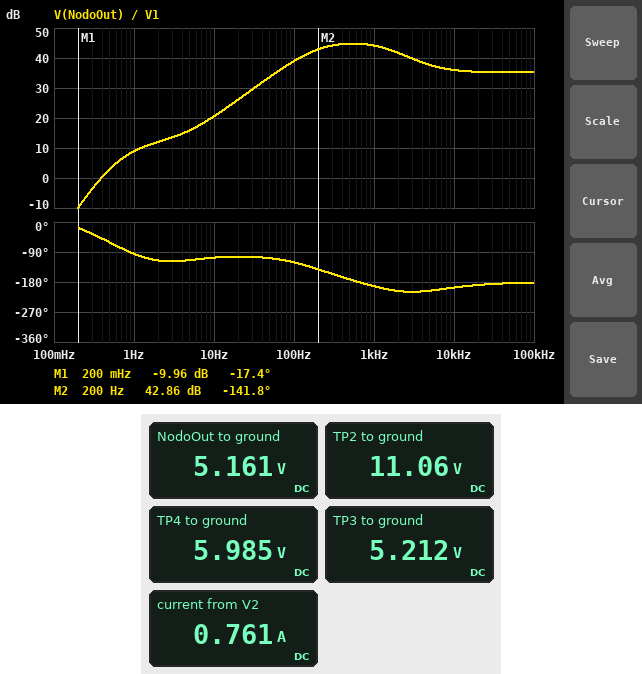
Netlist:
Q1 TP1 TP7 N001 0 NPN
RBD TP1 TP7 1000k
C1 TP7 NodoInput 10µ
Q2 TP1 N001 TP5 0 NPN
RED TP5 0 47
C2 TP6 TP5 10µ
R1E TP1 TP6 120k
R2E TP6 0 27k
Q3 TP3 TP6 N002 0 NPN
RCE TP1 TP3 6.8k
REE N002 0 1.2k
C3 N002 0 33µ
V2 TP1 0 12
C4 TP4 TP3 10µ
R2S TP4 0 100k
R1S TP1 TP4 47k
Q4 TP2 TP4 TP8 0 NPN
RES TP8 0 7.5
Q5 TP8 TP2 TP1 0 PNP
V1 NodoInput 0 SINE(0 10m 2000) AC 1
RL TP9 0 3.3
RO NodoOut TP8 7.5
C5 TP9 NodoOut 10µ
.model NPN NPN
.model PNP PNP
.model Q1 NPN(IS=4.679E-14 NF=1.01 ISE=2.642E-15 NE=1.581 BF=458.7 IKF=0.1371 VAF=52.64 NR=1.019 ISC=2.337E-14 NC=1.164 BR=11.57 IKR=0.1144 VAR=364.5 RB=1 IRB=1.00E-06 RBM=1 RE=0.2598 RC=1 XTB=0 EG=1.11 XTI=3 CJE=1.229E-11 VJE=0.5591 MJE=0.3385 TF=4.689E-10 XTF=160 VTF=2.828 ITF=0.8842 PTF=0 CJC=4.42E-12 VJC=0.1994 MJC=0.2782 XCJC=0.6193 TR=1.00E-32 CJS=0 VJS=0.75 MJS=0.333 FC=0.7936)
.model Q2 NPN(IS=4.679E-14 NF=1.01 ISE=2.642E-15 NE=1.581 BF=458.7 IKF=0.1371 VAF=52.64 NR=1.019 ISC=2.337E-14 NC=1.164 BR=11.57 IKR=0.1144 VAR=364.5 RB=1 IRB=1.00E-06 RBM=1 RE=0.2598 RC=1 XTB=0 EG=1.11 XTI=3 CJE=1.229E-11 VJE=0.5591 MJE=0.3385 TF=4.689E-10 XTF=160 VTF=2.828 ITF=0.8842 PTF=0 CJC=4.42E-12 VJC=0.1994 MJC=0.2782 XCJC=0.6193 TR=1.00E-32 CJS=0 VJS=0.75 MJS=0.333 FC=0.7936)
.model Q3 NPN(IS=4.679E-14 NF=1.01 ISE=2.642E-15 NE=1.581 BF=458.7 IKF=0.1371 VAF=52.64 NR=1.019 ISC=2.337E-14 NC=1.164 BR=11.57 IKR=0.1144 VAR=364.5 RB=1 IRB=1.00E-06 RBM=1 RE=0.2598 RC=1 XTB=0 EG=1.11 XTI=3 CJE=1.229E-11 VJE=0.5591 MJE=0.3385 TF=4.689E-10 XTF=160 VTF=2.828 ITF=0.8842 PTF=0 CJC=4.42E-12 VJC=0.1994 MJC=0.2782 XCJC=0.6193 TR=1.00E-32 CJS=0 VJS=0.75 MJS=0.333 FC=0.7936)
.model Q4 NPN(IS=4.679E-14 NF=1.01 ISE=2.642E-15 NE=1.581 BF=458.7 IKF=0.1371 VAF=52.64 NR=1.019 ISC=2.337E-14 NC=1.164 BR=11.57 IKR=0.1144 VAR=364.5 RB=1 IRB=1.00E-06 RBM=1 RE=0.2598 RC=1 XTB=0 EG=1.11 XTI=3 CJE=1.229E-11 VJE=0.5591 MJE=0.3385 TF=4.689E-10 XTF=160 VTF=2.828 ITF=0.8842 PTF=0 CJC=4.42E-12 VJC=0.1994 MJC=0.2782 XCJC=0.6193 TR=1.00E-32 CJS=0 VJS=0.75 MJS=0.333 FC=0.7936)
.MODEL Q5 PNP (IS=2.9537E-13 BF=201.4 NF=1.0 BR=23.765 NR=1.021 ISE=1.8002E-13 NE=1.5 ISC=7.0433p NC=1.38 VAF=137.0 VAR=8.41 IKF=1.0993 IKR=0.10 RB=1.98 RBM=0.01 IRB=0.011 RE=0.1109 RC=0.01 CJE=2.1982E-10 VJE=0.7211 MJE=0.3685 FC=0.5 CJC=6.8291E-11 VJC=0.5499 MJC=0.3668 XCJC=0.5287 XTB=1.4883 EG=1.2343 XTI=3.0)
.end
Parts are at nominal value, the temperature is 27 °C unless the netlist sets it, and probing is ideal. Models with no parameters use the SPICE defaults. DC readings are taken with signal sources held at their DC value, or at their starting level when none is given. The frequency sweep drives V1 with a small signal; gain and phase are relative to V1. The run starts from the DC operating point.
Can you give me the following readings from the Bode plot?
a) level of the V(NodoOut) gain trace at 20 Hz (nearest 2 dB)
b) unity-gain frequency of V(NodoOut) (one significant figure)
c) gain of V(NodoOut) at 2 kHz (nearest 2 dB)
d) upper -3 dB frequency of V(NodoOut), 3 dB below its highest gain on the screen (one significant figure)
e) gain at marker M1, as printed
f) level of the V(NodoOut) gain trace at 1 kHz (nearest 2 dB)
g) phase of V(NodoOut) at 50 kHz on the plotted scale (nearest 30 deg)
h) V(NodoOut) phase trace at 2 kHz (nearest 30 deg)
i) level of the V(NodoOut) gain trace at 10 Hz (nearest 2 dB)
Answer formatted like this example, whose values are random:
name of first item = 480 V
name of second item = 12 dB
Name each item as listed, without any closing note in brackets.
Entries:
level of the V(NodoOut) gain trace at 20 Hz = 26 dB
unity-gain frequency of V(NodoOut) = 400 mHz
gain of V(NodoOut) at 2 kHz = 42 dB
upper -3 dB frequency of V(NodoOut), 3 dB below its highest gain on the screen = 2 kHz
gain at marker M1, as printed = -9.96 dB
level of the V(NodoOut) gain trace at 1 kHz = 44 dB
phase of V(NodoOut) at 50 kHz on the plotted scale = -180 deg
V(NodoOut) phase trace at 2 kHz = -210 deg
level of the V(NodoOut) gain trace at 10 Hz = 20 dB
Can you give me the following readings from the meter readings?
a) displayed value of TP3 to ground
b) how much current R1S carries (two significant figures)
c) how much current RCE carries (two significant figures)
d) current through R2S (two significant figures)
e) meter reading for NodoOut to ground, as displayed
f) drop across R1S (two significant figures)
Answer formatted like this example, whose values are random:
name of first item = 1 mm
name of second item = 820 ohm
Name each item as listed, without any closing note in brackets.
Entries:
displayed value of TP3 to ground = 5.212 V
how much current R1S carries = 130 µA
how much current RCE carries = 1.0 mA
current through R2S = 60 µA
meter reading for NodoOut to ground, as displayed = 5.161 V
drop across R1S = 6.0 V
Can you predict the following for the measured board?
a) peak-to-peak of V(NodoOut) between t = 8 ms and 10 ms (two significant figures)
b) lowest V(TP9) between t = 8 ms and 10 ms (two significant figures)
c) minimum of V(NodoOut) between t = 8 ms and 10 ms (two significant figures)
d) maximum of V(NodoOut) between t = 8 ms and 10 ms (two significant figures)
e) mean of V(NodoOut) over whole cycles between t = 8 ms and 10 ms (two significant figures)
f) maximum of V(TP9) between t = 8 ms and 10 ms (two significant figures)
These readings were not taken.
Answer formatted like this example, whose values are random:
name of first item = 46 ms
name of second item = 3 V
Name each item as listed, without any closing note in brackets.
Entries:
peak-to-peak of V(NodoOut) between t = 8 ms and 10 ms = 2.4 V
lowest V(TP9) between t = 8 ms and 10 ms = -500 mV
minimum of V(NodoOut) between t = 8 ms and 10 ms = 3.9 V
maximum of V(NodoOut) between t = 8 ms and 10 ms = 6.3 V
mean of V(NodoOut) over whole cycles between t = 8 ms and 10 ms = 5.2 V
maximum of V(TP9) between t = 8 ms and 10 ms = 430 mV
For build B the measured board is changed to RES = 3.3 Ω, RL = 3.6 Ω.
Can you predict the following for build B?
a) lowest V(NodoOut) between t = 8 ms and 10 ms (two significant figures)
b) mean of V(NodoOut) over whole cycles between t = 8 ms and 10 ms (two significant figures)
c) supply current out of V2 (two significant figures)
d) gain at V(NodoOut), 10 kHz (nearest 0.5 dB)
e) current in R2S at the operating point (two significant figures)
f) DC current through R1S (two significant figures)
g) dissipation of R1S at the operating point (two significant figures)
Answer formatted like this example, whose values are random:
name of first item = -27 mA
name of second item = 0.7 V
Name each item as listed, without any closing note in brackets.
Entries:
lowest V(NodoOut) between t = 8 ms and 10 ms = 2.6 V
mean of V(NodoOut) over whole cycles between t = 8 ms and 10 ms = 3.7 V
supply current out of V2 = 1.2 A
gain at V(NodoOut), 10 kHz = 35.5 dB
current in R2S at the operating point = 46 µA
DC current through R1S = 160 µA
dissipation of R1S at the operating point = 1.2 mW
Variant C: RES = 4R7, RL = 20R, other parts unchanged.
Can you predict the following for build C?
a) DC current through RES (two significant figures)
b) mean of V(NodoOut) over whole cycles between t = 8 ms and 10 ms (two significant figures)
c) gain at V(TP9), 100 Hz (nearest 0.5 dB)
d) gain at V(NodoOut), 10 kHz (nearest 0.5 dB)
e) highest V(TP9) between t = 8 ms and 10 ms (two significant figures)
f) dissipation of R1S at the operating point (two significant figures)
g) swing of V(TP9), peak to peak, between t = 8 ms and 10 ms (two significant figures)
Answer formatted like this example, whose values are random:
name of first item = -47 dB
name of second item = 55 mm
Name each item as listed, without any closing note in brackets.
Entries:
DC current through RES = 930 mA
mean of V(NodoOut) over whole cycles between t = 8 ms and 10 ms = 4.4 V
gain at V(TP9), 100 Hz = 20.5 dB
gain at V(NodoOut), 10 kHz = 42.5 dB
highest V(TP9) between t = 8 ms and 10 ms = 1.2 V
dissipation of R1S at the operating point = 980 µW
swing of V(TP9), peak to peak, between t = 8 ms and 10 ms = 2.6 V
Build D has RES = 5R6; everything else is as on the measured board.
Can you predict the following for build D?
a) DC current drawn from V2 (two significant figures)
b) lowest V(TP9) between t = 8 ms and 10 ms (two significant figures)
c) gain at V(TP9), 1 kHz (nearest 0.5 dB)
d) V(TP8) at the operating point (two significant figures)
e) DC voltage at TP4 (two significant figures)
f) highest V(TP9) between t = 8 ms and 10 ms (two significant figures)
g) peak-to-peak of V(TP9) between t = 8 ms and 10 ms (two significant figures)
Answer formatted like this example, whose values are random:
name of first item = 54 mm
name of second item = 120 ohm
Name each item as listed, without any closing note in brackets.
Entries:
DC current drawn from V2 = 910 mA
lowest V(TP9) between t = 8 ms and 10 ms = -490 mV
gain at V(TP9), 1 kHz = 30.0 dB
V(TP8) at the operating point = 4.7 V
DC voltage at TP4 = 5.5 V
highest V(TP9) between t = 8 ms and 10 ms = 420 mV
peak-to-peak of V(TP9) between t = 8 ms and 10 ms = 910 mV
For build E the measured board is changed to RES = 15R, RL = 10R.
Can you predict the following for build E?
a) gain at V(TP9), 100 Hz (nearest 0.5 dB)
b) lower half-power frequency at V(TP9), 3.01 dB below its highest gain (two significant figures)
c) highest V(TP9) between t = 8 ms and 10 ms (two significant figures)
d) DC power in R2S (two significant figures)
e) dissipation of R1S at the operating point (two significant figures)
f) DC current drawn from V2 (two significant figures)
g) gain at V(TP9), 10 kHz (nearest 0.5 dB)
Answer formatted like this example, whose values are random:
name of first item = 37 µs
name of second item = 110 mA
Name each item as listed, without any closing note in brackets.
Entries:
gain at V(TP9), 100 Hz = 15.0 dB
lower half-power frequency at V(TP9), 3.01 dB below its highest gain = 920 Hz
highest V(TP9) between t = 8 ms and 10 ms = 940 mV
DC power in R2S = 470 µW
dissipation of R1S at the operating point = 560 µW
DC current drawn from V2 = 480 mA
gain at V(TP9), 10 kHz = 41.0 dB
